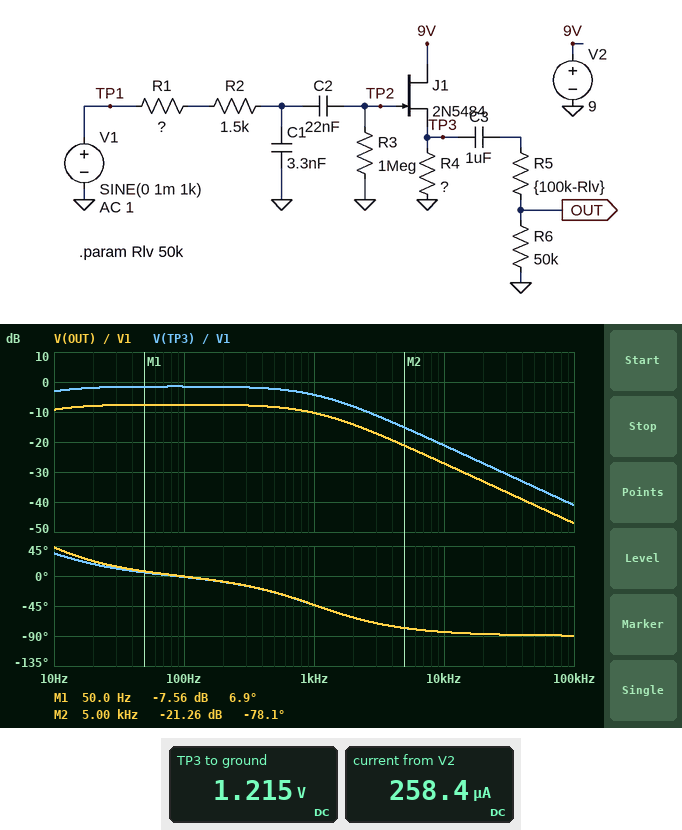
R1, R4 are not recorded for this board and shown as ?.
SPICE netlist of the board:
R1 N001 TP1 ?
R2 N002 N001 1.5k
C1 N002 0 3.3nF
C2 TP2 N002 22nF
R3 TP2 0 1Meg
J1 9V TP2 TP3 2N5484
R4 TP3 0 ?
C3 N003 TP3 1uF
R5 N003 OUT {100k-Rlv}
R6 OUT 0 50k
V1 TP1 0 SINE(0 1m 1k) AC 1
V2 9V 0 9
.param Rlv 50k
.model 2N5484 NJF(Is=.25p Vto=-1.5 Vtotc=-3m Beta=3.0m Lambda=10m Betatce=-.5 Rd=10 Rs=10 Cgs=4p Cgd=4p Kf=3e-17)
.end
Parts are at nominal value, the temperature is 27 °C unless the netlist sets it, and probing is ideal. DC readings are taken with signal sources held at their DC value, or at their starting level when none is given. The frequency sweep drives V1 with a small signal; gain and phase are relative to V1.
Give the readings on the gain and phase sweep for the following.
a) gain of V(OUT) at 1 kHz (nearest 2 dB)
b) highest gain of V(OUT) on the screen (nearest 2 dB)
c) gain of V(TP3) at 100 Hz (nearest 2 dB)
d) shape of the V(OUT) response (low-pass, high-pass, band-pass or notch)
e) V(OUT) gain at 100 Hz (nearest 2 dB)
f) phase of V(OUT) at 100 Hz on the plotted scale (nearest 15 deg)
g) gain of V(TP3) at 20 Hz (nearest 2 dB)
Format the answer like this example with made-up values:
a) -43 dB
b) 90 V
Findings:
a) -10 dB
b) -8 dB
c) -2 dB
d) low-pass
e) -8 dB
f) 0 deg
g) -2 dB
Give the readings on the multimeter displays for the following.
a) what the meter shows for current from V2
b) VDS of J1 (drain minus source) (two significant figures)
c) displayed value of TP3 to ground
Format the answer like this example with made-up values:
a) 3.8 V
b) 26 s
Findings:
a) 258.4 µA
b) 7.8 V
c) 1.215 V
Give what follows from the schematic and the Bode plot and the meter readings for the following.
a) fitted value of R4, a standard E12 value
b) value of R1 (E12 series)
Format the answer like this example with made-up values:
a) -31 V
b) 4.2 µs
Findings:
a) 4.7 kΩ
b) 47 kΩ
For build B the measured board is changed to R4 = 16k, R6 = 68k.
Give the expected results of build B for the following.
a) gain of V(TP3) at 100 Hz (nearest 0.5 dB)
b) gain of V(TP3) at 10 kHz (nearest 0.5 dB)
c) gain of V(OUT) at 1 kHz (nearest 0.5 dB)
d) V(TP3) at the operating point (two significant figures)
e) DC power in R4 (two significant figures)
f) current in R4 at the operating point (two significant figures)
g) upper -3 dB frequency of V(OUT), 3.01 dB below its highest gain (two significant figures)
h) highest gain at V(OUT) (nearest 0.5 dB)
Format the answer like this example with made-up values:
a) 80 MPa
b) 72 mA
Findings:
a) -1.0 dB
b) -20.5 dB
c) -8.5 dB
d) 1.3 V
e) 110 µW
f) 84 µA
g) 1.1 kHz
h) -6.0 dB
